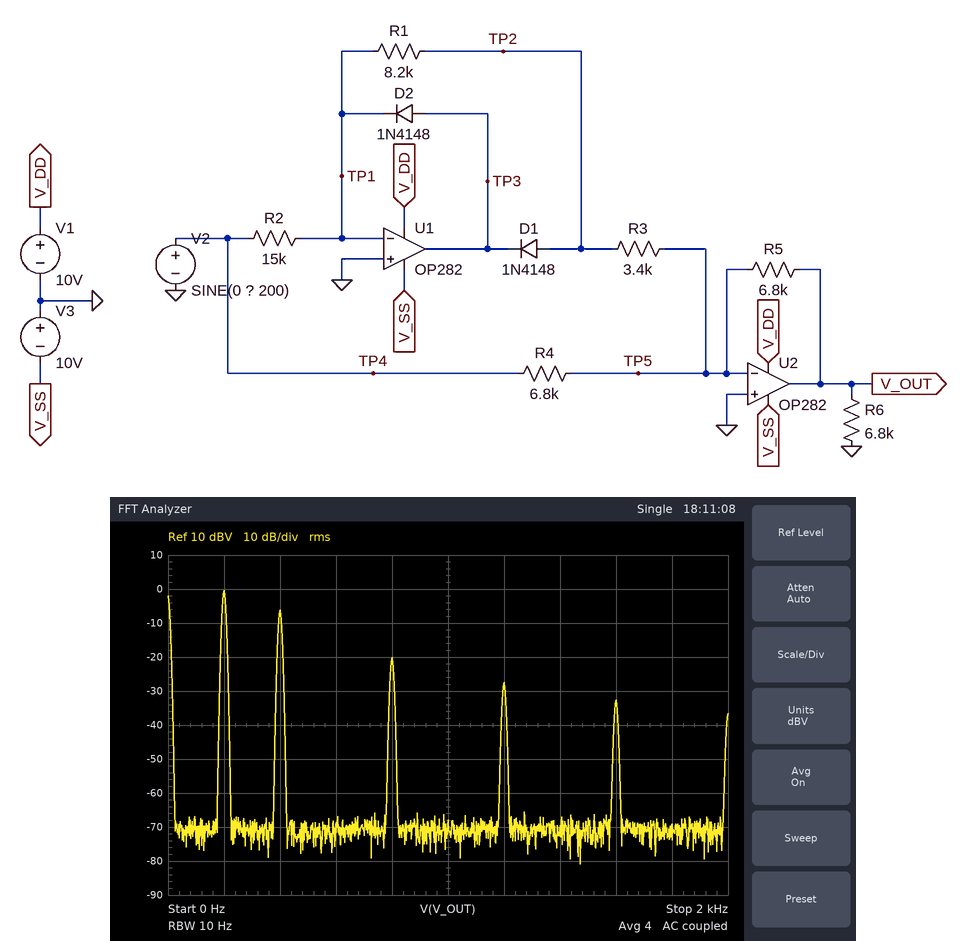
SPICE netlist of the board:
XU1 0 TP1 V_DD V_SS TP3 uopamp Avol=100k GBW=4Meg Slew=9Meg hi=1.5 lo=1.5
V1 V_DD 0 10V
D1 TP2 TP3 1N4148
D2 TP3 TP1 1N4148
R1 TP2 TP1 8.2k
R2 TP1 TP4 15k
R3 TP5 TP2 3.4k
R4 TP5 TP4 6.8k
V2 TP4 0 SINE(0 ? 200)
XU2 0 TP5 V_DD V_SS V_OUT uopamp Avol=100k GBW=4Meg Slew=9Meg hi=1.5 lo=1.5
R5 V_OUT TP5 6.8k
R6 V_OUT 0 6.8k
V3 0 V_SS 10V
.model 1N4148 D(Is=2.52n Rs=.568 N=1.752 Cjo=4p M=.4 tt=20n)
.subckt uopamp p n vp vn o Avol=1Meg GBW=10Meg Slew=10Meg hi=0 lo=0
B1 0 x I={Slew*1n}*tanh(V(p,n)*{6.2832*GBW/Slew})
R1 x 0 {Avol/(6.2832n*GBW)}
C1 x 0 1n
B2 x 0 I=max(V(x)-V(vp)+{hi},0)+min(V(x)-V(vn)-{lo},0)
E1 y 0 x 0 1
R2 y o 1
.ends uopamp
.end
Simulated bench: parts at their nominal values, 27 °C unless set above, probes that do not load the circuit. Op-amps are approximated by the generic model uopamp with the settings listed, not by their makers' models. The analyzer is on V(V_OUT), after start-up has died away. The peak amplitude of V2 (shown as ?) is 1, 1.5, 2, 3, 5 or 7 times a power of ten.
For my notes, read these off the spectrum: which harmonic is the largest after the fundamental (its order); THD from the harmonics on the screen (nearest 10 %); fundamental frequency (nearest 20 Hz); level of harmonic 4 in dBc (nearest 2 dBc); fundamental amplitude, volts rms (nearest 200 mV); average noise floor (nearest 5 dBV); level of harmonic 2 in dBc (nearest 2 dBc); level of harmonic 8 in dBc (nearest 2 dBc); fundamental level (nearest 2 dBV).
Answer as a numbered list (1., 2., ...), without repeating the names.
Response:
1. 2
2. 50 %
3. 200 Hz
4. -20 dBc
5. 1.0 V
6. -70 dBV
7. -6 dBc
8. -32 dBc
9. 0 dBV
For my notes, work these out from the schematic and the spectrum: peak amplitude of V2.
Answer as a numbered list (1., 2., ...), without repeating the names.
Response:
1. 3 V
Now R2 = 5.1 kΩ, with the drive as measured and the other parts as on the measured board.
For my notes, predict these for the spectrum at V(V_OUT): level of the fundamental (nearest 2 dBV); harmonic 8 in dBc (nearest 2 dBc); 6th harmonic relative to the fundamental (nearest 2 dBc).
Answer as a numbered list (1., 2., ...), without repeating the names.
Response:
1. 2 dBV
2. -26 dBc
3. -20 dBc
